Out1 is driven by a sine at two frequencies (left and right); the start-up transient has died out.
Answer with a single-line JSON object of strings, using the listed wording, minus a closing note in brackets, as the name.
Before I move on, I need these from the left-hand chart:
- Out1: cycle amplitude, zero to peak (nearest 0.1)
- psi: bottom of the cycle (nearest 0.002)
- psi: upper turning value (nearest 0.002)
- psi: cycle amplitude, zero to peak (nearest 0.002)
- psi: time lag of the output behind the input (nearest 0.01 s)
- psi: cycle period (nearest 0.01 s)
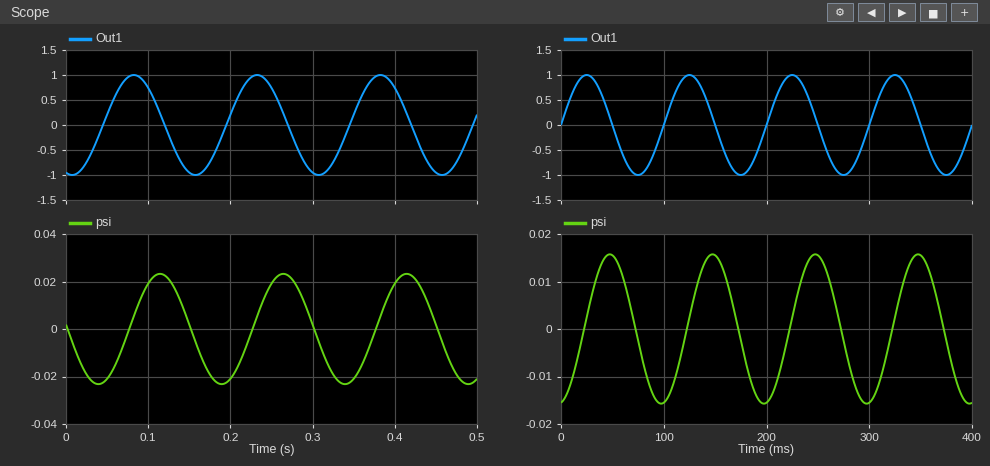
{"Out1: cycle amplitude, zero to peak": "1.0", "psi: bottom of the cycle": "-0.024", "psi: upper turning value": "0.024", "psi: cycle amplitude, zero to peak": "0.024", "psi: time lag of the output behind the input": "0.03 s", "psi: cycle period": "0.15 s"}
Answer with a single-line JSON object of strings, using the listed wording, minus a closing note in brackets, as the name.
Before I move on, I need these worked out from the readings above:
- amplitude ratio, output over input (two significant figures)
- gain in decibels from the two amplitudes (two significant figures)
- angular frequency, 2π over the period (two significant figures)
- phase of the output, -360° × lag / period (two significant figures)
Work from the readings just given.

{"amplitude ratio, output over input": "0.024", "gain in decibels from the two amplitudes": "-32 dB", "angular frequency, 2π over the period": "42 rad/s", "phase of the output, -360° × lag / period": "-72°"}
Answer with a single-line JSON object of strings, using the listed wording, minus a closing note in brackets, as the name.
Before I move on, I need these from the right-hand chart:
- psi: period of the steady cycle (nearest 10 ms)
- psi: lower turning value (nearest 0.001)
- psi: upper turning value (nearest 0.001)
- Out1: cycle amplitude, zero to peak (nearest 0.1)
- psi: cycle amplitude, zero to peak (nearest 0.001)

{"psi: period of the steady cycle": "100 ms", "psi: lower turning value": "-0.016", "psi: upper turning value": "0.016", "Out1: cycle amplitude, zero to peak": "1.0", "psi: cycle amplitude, zero to peak": "0.016"}
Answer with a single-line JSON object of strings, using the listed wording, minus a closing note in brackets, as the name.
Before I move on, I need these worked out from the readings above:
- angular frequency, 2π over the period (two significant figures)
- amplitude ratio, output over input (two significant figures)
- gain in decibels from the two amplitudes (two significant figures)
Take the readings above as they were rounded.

{"angular frequency, 2π over the period": "0.063 rad/ms", "amplitude ratio, output over input": "0.016", "gain in decibels from the two amplitudes": "-36 dB"}
